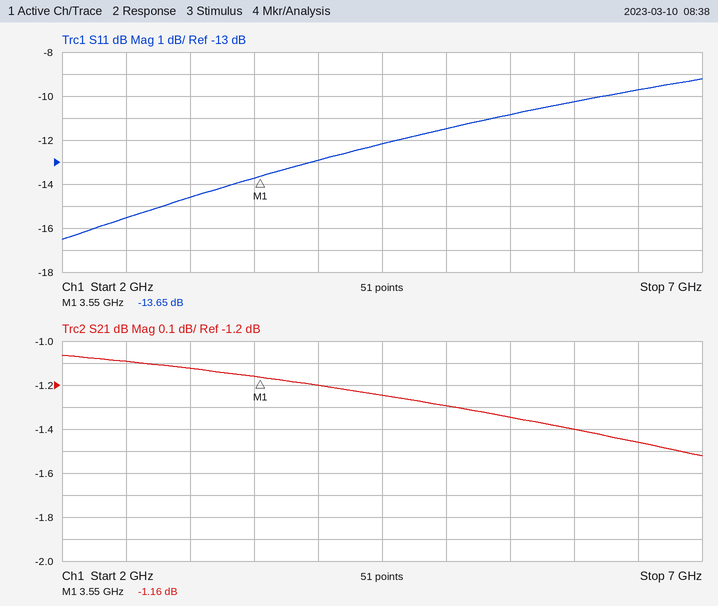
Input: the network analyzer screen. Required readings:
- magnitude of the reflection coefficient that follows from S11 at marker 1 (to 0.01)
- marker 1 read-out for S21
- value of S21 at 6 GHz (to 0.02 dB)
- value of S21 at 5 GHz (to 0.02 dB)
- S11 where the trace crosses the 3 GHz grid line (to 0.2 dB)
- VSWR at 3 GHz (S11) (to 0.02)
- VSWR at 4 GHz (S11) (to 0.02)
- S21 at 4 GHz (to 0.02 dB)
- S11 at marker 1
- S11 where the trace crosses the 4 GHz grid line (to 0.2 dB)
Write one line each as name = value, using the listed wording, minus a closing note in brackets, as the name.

magnitude of the reflection coefficient that follows from S11 at marker 1 = 0.21
marker 1 read-out for S21 = -1.16 dB
value of S21 at 6 GHz = -1.40 dB
value of S21 at 5 GHz = -1.30 dB
S11 where the trace crosses the 3 GHz grid line = -14.6 dB
VSWR at 3 GHz (S11) = 1.46
VSWR at 4 GHz (S11) = 1.58
S21 at 4 GHz = -1.20 dB
S11 at marker 1 = -13.65 dB
S11 where the trace crosses the 4 GHz grid line = -13.0 dB
